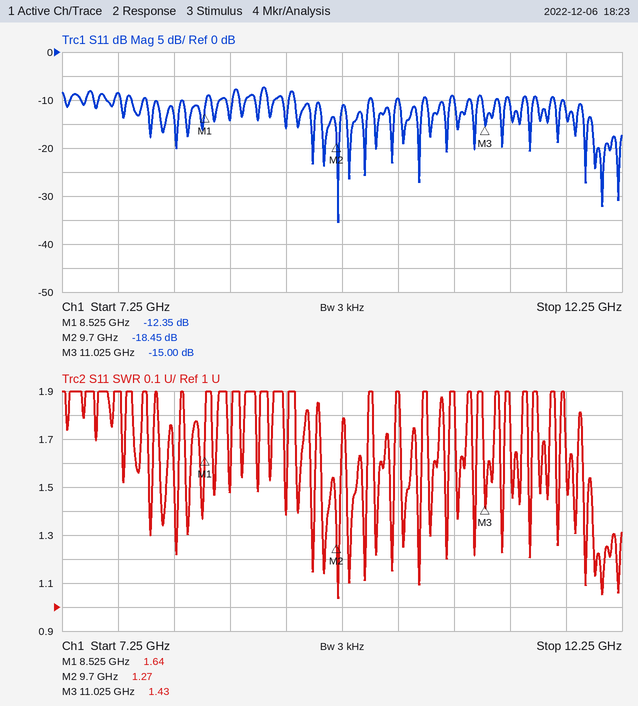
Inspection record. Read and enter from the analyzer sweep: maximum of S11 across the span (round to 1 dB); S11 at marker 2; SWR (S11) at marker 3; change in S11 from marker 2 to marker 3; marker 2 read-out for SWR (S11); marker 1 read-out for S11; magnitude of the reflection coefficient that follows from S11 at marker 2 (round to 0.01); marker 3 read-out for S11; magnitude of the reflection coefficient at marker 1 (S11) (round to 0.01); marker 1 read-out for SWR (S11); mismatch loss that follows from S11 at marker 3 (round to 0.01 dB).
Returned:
-7 dB
-18.45 dB
1.43
3.45 dB
1.27
-12.35 dB
0.12
-15.00 dB
0.24
1.64
0.14 dB
